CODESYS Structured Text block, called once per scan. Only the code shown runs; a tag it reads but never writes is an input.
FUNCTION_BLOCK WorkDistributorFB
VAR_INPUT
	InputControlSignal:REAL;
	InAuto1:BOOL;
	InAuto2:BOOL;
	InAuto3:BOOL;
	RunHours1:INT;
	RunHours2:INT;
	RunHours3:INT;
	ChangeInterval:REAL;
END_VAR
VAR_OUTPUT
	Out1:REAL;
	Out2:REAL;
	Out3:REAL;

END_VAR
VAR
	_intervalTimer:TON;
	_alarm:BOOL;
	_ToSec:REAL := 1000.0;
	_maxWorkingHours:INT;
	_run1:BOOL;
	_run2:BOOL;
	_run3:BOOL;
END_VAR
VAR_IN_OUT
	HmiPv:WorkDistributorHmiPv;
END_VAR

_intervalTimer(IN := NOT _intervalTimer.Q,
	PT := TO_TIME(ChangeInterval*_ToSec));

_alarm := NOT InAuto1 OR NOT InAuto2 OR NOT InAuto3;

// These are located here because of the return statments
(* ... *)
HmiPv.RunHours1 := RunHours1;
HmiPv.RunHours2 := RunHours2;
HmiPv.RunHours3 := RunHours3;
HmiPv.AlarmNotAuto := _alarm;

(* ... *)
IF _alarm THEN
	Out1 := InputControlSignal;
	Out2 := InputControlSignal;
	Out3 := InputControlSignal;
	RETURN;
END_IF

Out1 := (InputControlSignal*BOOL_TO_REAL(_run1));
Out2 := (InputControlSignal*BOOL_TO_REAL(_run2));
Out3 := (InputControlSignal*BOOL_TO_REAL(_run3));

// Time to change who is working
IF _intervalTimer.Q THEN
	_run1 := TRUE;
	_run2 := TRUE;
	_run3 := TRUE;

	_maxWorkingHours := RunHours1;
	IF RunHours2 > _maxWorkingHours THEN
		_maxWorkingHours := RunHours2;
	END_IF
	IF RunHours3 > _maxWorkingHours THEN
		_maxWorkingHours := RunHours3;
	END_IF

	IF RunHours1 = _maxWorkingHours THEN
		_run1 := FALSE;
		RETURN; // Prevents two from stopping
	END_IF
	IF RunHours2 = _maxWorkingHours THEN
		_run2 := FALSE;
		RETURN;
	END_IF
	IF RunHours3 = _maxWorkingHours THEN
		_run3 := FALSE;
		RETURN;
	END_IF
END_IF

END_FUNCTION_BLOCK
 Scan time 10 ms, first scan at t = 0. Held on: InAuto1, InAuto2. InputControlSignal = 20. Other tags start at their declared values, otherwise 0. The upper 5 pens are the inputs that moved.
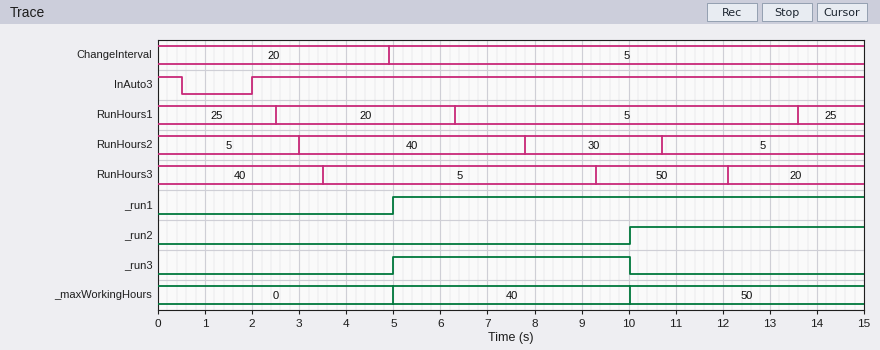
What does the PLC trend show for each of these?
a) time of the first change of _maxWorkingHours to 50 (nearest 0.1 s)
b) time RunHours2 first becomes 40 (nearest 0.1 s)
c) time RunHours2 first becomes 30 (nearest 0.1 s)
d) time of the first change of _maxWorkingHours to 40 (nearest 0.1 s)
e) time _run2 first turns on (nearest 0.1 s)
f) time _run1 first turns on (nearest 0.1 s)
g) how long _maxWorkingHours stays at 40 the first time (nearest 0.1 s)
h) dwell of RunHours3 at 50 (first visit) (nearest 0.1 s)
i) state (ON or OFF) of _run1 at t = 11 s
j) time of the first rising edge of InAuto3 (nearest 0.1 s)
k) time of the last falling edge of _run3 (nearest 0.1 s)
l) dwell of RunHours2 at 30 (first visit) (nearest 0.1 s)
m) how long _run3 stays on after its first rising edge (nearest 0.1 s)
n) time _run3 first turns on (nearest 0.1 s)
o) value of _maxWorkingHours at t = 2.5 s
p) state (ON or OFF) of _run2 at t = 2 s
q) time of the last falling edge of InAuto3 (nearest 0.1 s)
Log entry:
10.0 s
3.0 s
7.8 s
5.0 s
10.0 s
5.0 s
5.0 s
2.8 s
ON
2.0 s
10.0 s
2.9 s
5.0 s
5.0 s
0
OFF
0.5 s
